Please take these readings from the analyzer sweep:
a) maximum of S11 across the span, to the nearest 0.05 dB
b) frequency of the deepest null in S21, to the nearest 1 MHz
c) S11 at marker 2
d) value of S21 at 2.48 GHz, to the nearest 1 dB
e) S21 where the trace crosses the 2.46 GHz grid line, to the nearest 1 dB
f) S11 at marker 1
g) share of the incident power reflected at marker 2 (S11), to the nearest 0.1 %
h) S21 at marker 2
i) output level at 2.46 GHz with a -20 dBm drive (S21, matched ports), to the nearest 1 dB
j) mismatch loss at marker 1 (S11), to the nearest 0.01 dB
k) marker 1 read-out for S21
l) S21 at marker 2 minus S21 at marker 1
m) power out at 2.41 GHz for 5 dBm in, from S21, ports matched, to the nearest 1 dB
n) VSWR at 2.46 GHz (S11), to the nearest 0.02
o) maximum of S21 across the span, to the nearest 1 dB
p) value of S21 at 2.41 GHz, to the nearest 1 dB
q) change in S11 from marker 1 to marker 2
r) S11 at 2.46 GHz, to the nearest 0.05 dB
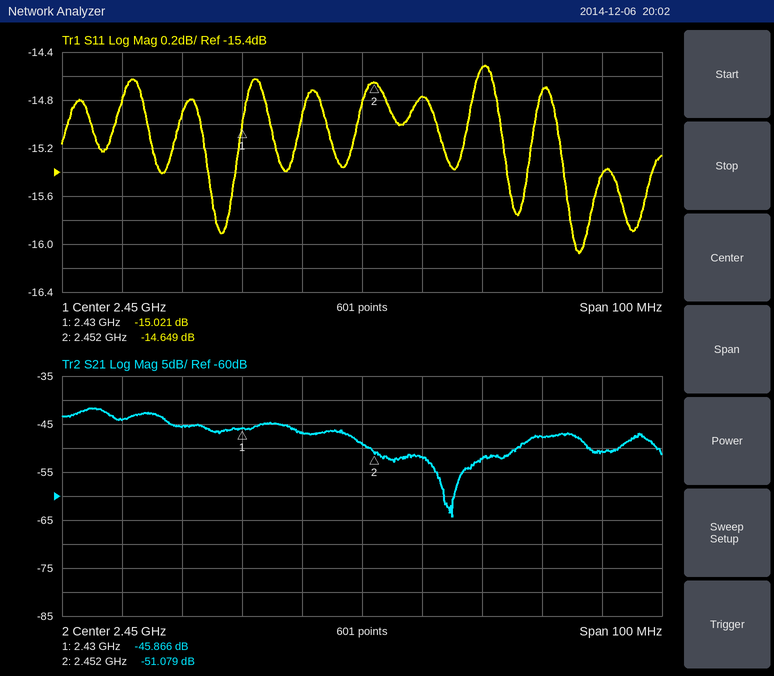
-14.50 dB
2.465 GHz
-14.649 dB
-48 dB
-52 dB
-15.021 dB
3.4 %
-51.079 dB
-72 dBm
0.14 dB
-45.866 dB
-5.213 dB
-39 dBm
1.44
-42 dB
-44 dB
0.372 dB
-14.75 dB
